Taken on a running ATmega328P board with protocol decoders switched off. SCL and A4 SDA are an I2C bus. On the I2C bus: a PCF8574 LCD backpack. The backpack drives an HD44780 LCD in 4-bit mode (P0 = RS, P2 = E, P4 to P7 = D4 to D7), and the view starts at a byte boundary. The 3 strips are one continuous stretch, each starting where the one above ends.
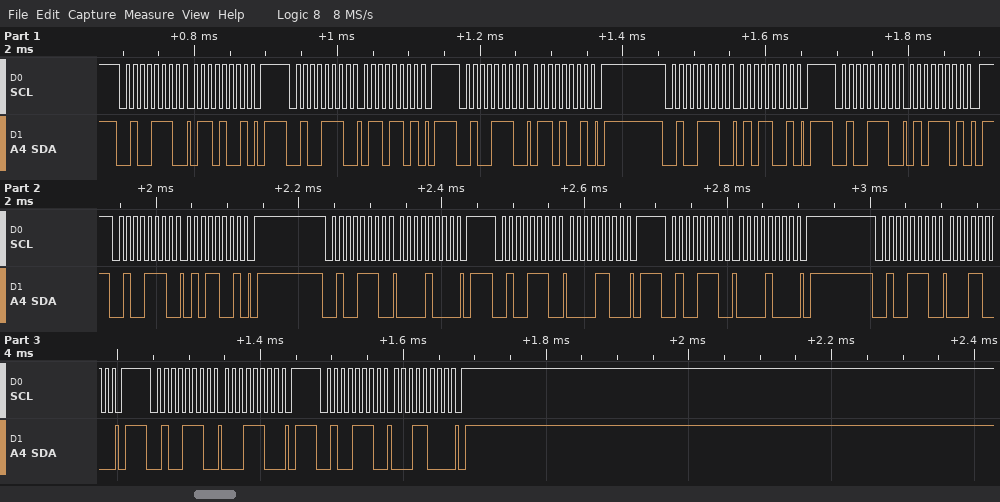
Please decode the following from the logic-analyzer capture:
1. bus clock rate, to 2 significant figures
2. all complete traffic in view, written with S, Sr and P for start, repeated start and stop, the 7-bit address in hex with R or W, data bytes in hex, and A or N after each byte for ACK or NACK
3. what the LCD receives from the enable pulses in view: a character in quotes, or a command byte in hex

100 kHz
S 27W A 69 A P S 27W A 6D A P S 27W A 69 A P S 27W A 59 A P S 27W A 5D A P S 27W A 59 A P S 27W A 08 A P S 27W A 0C A P S 27W A 08 A P S 27W A 18 A P S 27W A 1C A P S 27W A 18 A P
'e' 0x01
